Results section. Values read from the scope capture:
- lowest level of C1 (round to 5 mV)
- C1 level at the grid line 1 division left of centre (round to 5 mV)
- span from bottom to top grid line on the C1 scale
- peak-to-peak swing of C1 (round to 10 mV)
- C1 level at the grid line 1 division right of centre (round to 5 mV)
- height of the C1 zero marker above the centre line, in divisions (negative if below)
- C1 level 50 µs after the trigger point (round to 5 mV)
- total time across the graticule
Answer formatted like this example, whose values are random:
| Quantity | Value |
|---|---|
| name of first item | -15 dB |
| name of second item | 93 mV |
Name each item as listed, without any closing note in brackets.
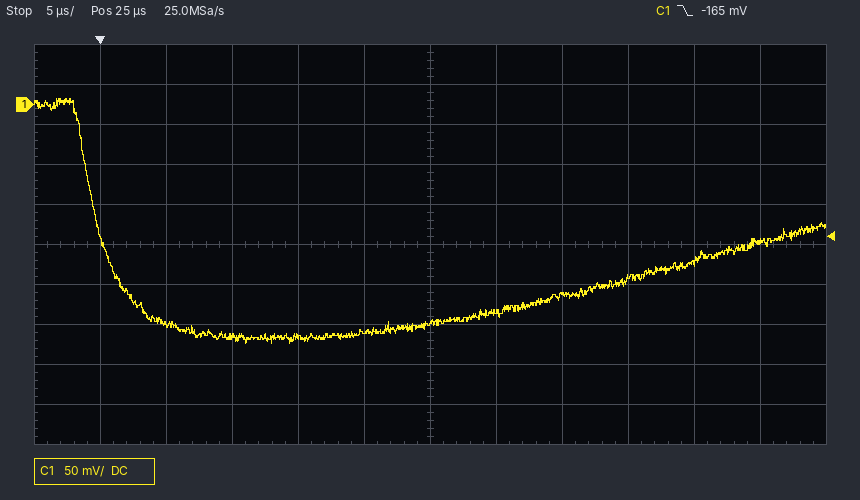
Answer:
| Quantity | Value |
|---|---|
| lowest level of C1 | -300 mV |
| C1 level at the grid line 1 division left of centre | -285 mV |
| span from bottom to top grid line on the C1 scale | 500 mV |
| peak-to-peak swing of C1 | 310 mV |
| C1 level at the grid line 1 division right of centre | -260 mV |
| height of the C1 zero marker above the centre line, in divisions | +3.5 div |
| C1 level 50 µs after the trigger point | -170 mV |
| total time across the graticule | 60 µs |
